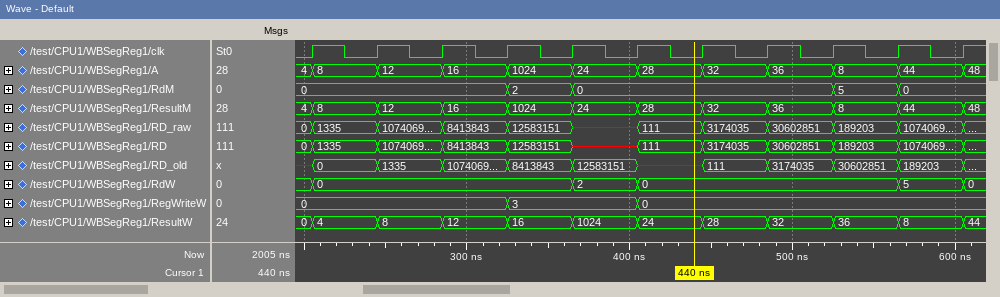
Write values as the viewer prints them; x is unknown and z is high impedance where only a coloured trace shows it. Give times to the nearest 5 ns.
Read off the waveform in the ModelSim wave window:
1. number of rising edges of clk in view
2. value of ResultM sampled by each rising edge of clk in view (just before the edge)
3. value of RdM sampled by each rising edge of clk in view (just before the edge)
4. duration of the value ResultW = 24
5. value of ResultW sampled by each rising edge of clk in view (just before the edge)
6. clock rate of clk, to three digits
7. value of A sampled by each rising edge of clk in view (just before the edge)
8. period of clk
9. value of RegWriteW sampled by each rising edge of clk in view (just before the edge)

11
4, 8, 12, 16, 1024, 24, 28, 32, 36, 8, 44
0, 0, 0, 0, 2, 0, 0, 0, 0, 5, 0
40 ns
0, 4, 8, 12, 16, 1024, 24, 28, 32, 36, 8
25.0 MHz
4, 8, 12, 16, 1024, 24, 28, 32, 36, 8, 44
40 ns
0, 0, 0, 0, 3, 3, 0, 0, 0, 0, 0
